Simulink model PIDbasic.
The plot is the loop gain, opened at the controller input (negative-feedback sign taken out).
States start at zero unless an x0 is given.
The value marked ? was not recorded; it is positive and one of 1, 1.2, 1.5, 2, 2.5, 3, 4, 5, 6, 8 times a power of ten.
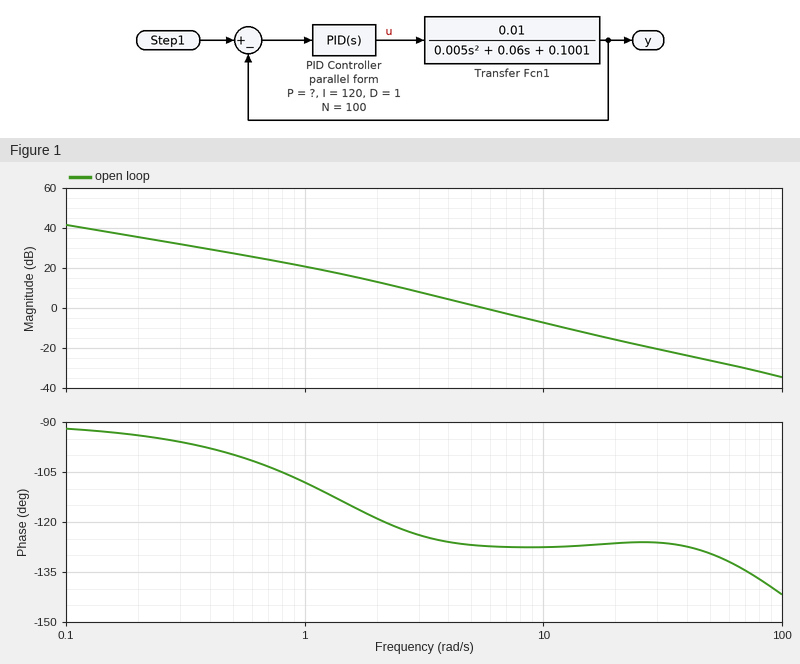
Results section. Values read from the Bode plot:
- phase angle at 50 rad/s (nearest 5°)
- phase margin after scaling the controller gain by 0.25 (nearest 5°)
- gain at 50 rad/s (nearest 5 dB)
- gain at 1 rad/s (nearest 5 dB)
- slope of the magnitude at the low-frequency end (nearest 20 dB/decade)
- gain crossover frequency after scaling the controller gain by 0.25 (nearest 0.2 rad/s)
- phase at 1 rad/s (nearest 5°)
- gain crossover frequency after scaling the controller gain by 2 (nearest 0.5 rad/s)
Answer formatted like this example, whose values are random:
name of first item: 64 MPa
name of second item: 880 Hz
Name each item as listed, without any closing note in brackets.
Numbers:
phase angle at 50 rad/s: -130°
phase margin after scaling the controller gain by 0.25: 60°
gain at 50 rad/s: -25 dB
gain at 1 rad/s: 20 dB
slope of the magnitude at the low-frequency end: -20 dB/decade
gain crossover frequency after scaling the controller gain by 0.25: 2.2 rad/s
phase at 1 rad/s: -110°
gain crossover frequency after scaling the controller gain by 2: 9.0 rad/s
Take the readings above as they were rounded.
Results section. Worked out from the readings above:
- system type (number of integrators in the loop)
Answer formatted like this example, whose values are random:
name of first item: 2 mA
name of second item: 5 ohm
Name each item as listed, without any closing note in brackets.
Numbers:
system type: 1
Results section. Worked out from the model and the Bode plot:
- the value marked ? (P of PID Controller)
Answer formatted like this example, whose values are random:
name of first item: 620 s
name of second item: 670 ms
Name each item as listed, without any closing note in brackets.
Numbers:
the value marked ?: 30
